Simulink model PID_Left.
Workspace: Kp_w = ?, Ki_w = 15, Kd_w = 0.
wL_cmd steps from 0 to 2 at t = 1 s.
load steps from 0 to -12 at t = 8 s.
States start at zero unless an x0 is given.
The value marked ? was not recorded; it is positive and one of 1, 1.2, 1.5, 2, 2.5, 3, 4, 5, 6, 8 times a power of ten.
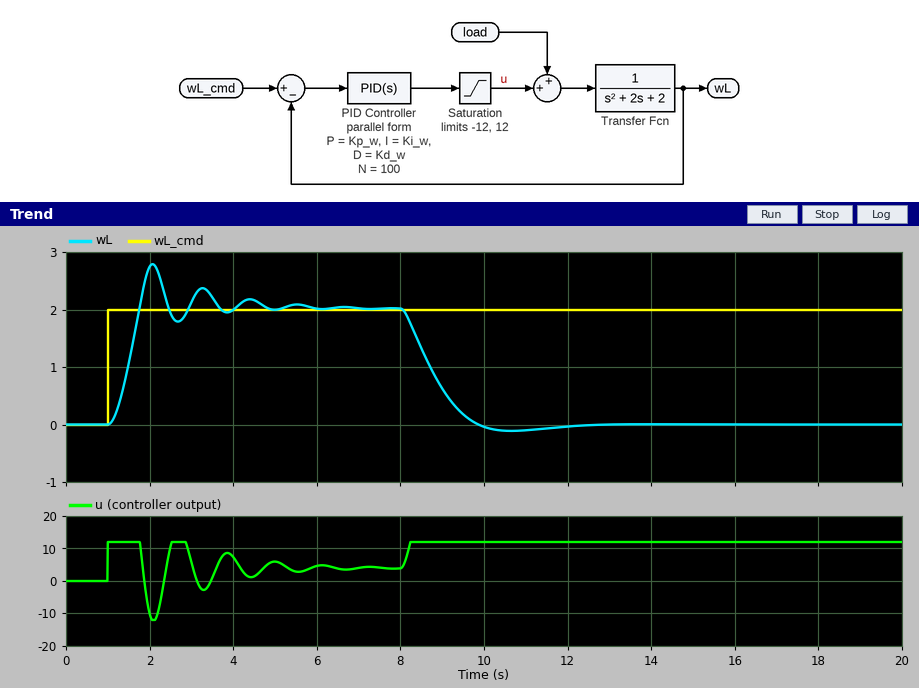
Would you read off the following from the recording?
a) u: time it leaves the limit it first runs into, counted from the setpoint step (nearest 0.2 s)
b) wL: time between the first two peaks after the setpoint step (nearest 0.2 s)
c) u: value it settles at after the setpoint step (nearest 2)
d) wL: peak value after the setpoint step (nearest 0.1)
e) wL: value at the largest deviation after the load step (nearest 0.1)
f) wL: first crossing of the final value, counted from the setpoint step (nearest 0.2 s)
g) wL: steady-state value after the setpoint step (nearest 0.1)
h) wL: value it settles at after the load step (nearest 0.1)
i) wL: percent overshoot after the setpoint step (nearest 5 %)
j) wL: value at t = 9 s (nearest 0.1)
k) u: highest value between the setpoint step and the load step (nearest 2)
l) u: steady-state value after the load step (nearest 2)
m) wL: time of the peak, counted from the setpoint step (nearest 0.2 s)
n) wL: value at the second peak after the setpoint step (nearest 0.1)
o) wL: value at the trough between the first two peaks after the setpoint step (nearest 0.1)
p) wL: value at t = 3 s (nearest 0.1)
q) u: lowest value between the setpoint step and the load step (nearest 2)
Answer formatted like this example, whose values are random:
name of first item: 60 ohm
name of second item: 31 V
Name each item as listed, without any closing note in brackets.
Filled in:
u: time it leaves the limit it first runs into, counted from the setpoint step: 0.8 s
wL: time between the first two peaks after the setpoint step: 1.2 s
u: value it settles at after the setpoint step: 4
wL: peak value after the setpoint step: 2.8
wL: value at the largest deviation after the load step: -0.1
wL: first crossing of the final value, counted from the setpoint step: 0.8 s
wL: steady-state value after the setpoint step: 2.0
wL: value it settles at after the load step: 0.0
wL: percent overshoot after the setpoint step: 40 %
wL: value at t = 9 s: 0.6
u: highest value between the setpoint step and the load step: 12
u: steady-state value after the load step: 12
wL: time of the peak, counted from the setpoint step: 1.0 s
wL: value at the second peak after the setpoint step: 2.4
wL: value at the trough between the first two peaks after the setpoint step: 1.8
wL: value at t = 3 s: 2.1
u: lowest value between the setpoint step and the load step: -12
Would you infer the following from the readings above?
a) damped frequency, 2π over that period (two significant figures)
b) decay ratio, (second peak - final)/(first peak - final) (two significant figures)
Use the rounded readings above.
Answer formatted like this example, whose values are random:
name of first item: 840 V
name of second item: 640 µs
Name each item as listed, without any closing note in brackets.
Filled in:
damped frequency, 2π over that period: 5.2 rad/s
decay ratio, (second peak - final)/(first peak - final): 0.50
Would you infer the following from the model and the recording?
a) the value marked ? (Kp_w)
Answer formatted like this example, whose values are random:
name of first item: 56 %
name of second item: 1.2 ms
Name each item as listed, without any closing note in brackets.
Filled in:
the value marked ?: 30
